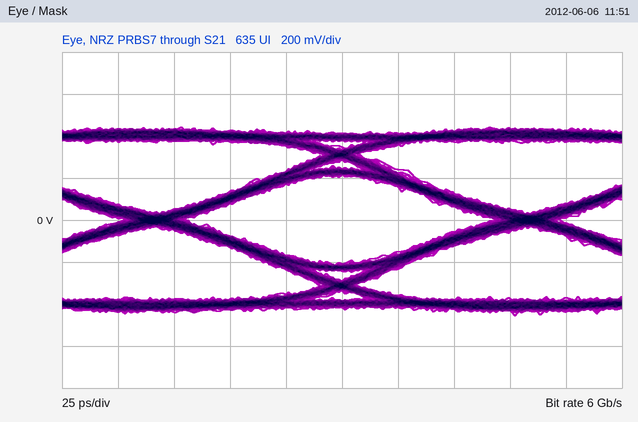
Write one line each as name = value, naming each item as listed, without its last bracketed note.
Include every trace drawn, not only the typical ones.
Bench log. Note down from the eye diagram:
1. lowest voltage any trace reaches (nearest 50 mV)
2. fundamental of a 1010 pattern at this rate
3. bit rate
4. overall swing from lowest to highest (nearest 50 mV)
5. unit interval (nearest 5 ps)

lowest voltage any trace reaches = -450 mV
fundamental of a 1010 pattern at this rate = 3 GHz
bit rate = 6 Gb/s
overall swing from lowest to highest = 900 mV
unit interval = 165 ps
